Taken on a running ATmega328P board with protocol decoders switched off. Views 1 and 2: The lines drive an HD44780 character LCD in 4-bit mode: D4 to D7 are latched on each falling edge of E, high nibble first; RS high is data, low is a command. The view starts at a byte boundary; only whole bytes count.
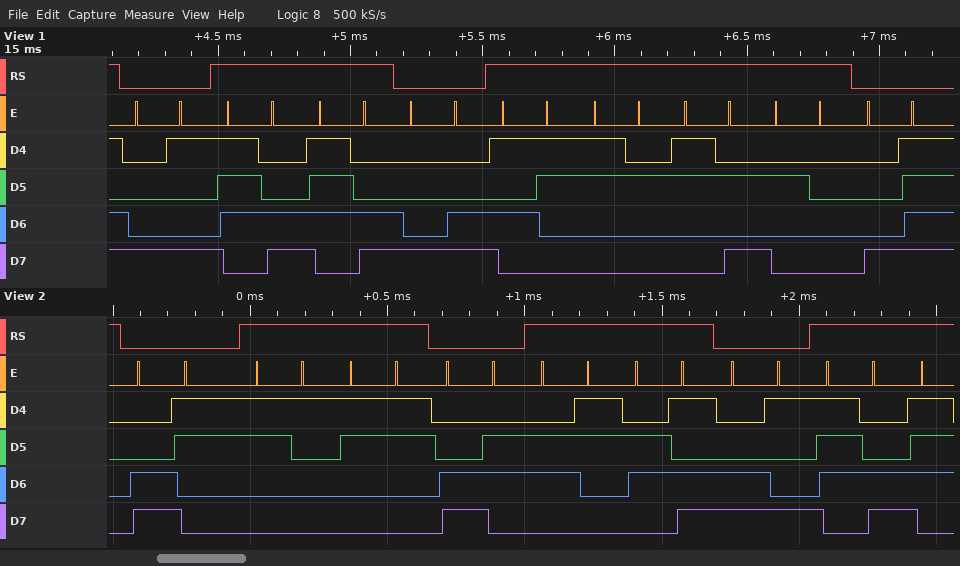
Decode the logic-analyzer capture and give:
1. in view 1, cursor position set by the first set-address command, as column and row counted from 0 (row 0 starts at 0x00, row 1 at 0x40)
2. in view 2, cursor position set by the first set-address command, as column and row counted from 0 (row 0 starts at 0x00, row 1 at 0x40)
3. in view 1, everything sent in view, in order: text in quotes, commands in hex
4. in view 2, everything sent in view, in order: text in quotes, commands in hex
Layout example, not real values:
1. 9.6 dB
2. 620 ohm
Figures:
1. column 9, row 0
2. column 3, row 1
3. 0x89 "||" 0x8C "S2: " 0x8F
4. 0xC3 "13" 0xC6 "cm" 0xC9 "|"
